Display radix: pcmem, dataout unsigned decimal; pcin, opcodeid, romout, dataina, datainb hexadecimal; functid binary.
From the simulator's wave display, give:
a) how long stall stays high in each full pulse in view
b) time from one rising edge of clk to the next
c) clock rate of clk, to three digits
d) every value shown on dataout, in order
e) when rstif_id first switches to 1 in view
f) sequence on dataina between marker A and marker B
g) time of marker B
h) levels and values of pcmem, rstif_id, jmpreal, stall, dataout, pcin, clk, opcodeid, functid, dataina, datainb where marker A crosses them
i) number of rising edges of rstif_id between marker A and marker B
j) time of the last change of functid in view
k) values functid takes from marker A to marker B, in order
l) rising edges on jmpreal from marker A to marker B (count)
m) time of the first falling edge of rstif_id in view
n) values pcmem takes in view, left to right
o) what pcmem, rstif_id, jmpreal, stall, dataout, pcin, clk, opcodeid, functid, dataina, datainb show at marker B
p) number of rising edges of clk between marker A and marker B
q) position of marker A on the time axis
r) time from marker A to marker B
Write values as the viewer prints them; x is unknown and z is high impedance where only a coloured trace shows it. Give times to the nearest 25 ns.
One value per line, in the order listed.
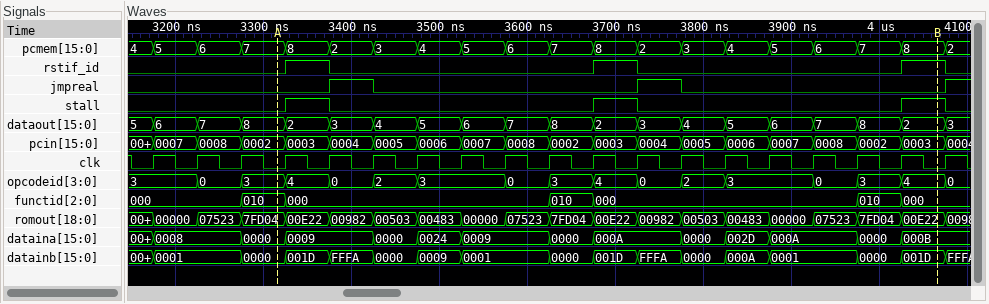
50 ns, 50 ns, 50 ns
50 ns
20.0 MHz
5, 6, 7, 8, 2, 3, 4, 5, 6, 7, 8, 2, 3, 4, 5, 6, 7, 8, 2, 3
3325 ns
0000, 0009, 0000, 0024, 0009, 0000, 000A, 0000, 002D, 000A, 0000, 000B
4075 ns
pcmem=7, rstif_id=0, jmpreal=0, stall=0, dataout=8, pcin=0002, clk=0, opcodeid=3, functid=010, dataina=0000, datainb=0000
3
4025 ns
010, 000, 010, 000, 010, 000
2
3375 ns
4, 5, 6, 7, 8, 2, 3, 4, 5, 6, 7, 8, 2, 3, 4, 5, 6, 7, 8, 2
pcmem=8, rstif_id=1, jmpreal=0, stall=1, dataout=2, pcin=0003, clk=0, opcodeid=4, functid=000, dataina=000B, datainb=001D
15
3325 ns
750 ns
